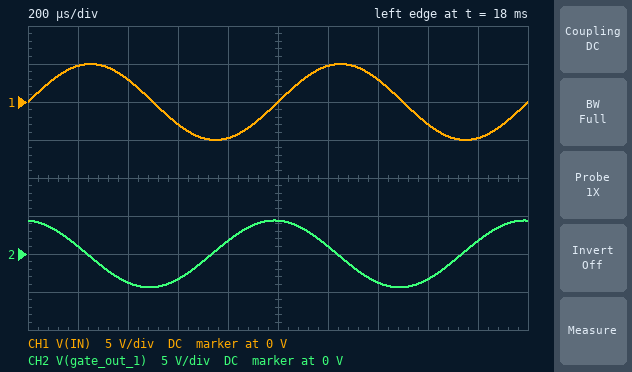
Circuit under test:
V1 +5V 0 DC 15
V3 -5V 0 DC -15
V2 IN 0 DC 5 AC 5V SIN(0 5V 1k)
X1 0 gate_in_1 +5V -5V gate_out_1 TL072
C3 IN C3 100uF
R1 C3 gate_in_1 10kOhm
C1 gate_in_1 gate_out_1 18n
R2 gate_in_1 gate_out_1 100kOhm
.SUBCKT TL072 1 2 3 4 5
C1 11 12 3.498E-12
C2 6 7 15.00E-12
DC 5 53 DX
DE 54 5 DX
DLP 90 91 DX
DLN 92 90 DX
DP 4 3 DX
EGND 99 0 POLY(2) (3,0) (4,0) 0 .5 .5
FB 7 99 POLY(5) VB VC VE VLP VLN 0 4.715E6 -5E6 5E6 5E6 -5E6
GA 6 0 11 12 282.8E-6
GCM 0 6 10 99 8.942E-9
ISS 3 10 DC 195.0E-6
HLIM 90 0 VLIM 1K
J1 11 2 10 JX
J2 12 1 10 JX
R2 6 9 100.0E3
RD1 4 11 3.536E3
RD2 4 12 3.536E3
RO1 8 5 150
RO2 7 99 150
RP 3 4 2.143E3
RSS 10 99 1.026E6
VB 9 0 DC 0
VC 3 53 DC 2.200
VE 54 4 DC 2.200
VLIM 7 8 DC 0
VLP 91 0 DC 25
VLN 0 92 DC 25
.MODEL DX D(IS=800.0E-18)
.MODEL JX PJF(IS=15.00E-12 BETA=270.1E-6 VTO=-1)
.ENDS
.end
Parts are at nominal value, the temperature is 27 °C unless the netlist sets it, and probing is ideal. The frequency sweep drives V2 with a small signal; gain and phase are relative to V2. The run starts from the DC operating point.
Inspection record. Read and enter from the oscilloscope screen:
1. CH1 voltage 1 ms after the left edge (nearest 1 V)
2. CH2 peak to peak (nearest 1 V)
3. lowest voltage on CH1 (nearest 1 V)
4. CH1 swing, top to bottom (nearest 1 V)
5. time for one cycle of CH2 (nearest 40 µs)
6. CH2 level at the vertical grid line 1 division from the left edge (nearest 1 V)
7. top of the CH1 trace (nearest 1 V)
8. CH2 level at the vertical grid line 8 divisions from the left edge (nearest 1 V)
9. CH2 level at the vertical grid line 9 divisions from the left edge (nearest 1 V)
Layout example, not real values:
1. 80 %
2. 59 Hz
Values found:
1. 0 V
2. 9 V
3. -5 V
4. 10 V
5. 1.00 ms
6. 1 V
7. 5 V
8. -3 V
9. 2 V
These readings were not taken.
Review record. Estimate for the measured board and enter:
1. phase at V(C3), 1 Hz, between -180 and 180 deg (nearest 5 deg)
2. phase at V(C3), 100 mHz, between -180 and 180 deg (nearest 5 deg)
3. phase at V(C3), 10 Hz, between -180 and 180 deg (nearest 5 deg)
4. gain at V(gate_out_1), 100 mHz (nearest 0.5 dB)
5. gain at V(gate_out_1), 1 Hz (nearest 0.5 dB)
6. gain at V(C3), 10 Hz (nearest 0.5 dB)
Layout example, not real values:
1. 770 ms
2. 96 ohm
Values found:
1. 10 deg
2. 60 deg
3. 0 deg
4. 14.5 dB
5. 20.0 dB
6. 0 dB
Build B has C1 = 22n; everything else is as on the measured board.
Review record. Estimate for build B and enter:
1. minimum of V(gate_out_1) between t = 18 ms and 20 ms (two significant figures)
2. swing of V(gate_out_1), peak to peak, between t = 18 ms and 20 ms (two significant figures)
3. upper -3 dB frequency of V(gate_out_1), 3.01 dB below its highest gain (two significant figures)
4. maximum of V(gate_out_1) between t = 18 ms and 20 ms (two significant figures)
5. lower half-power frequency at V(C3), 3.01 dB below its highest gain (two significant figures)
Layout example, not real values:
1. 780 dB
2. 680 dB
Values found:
1. -3.6 V
2. 7.2 V
3. 73 Hz
4. 3.6 V
5. 160 mHz
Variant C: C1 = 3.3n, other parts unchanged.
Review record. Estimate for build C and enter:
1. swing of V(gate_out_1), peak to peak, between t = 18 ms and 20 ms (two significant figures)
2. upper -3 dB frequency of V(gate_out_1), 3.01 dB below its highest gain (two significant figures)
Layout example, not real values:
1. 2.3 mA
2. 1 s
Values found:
1. 27 V
2. 480 Hz
